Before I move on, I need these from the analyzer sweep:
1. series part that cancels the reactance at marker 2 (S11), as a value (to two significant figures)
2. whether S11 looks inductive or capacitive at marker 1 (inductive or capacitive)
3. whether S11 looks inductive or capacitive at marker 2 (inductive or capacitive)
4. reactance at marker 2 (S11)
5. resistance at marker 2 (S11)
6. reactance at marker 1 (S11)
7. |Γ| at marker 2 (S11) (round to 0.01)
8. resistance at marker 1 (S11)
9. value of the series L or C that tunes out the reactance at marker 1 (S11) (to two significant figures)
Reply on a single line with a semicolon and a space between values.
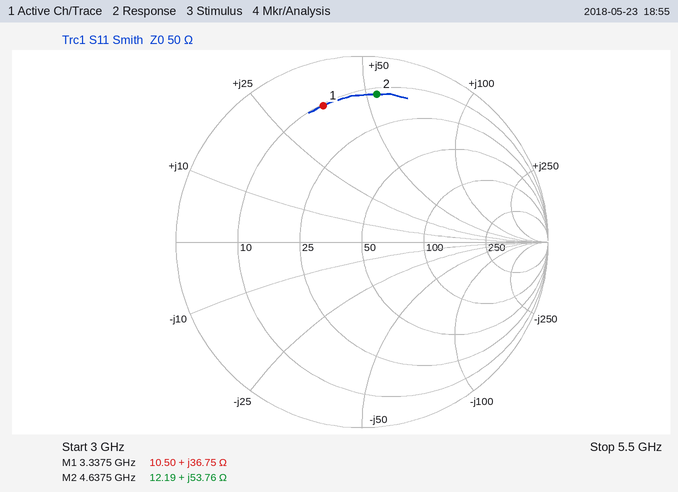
640 fF; inductive; inductive; +53.76 Ω; 12.19 Ω; +36.75 Ω; 0.80; 10.50 Ω; 1.3 pF
